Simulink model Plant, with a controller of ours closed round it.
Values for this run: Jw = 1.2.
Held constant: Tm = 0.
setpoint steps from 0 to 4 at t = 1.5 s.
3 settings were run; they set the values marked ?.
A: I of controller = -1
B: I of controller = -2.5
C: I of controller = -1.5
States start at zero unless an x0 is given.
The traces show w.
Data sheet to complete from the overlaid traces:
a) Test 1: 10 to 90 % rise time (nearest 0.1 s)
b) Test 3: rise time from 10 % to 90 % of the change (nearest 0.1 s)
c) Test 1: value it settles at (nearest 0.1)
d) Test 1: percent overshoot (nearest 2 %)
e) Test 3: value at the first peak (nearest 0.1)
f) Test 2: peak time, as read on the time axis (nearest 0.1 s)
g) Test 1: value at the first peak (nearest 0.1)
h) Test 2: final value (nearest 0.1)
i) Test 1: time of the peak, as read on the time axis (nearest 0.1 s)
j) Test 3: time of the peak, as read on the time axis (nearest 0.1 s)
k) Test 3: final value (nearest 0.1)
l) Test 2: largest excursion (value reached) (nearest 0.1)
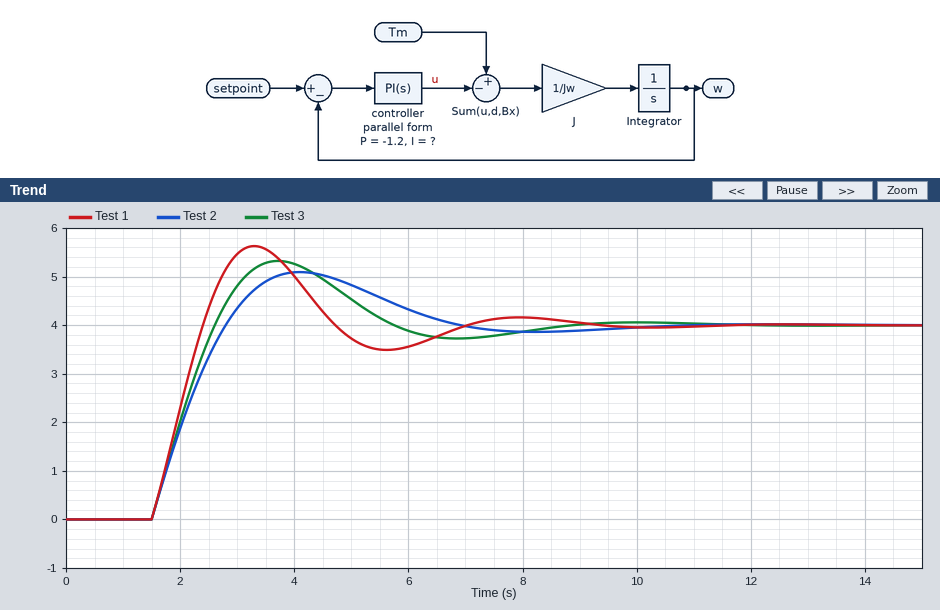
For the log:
0.7 s
0.9 s
4.0
40 %
5.3
4.1 s
5.6
4.0
3.3 s
3.7 s
4.0
5.1
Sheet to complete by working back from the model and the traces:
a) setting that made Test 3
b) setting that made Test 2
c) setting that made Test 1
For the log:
C
A
B
